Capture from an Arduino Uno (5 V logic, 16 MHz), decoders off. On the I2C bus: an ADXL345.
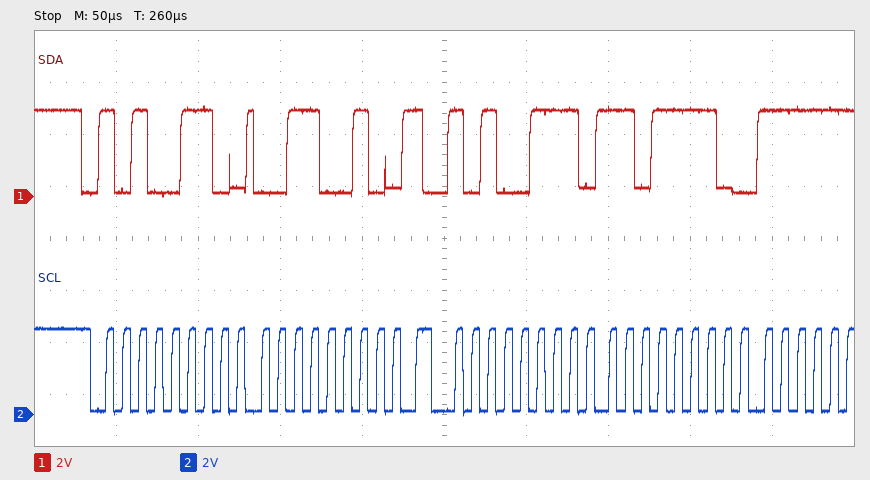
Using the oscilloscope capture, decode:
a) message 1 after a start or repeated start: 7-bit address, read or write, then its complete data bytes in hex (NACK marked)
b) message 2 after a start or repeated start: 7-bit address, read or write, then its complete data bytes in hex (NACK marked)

0x53 write: 32
0x53 read: DE
